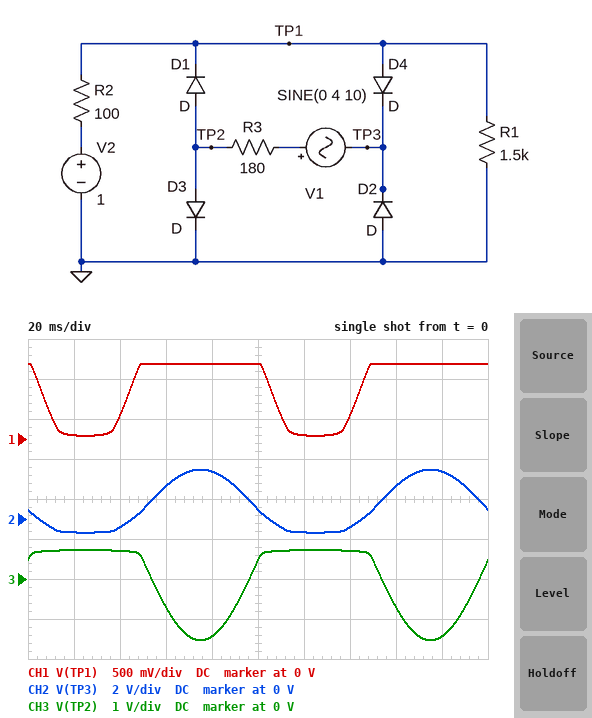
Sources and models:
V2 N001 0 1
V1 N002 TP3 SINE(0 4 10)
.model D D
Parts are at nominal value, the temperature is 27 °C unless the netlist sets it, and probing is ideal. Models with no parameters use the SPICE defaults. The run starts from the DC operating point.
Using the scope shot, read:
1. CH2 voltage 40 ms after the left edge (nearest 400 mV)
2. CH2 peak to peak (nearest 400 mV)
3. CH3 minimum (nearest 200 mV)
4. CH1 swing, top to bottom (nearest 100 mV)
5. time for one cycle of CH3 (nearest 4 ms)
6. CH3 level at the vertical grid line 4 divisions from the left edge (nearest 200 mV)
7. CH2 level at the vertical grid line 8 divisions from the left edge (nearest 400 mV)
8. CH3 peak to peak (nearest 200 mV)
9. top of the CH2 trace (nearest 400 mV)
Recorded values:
-400 mV
3.2 V
-1.6 V
900 mV
100 ms
-1.4 V
1.6 V
2.2 V
2.4 V
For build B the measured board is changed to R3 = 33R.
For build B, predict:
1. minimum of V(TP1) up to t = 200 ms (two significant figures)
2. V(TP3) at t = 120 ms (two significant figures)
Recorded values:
6.8 mV
-740 mV
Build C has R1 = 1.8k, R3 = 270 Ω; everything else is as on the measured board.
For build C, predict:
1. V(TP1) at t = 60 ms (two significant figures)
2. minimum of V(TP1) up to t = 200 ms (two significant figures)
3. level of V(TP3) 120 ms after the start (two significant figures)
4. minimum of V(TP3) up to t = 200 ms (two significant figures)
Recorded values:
950 mV
84 mV
-610 mV
-630 mV
